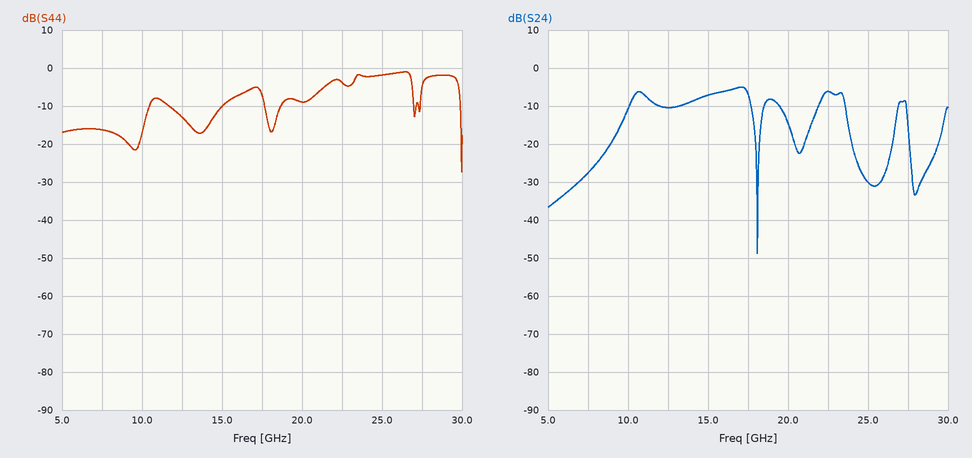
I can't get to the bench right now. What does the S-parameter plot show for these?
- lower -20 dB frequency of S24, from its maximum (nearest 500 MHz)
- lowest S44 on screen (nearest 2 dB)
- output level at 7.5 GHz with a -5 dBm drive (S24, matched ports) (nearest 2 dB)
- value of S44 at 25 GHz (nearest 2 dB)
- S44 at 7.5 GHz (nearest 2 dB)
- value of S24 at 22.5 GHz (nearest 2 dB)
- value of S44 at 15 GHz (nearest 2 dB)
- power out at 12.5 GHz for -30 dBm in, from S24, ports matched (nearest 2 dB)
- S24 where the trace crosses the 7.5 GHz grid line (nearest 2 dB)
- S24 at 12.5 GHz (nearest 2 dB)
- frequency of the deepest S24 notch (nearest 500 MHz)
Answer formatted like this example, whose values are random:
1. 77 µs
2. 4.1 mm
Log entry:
1. 8.0 GHz
2. -28 dB
3. -32 dBm
4. -2 dB
5. -16 dB
6. -6 dB
7. -10 dB
8. -40 dBm
9. -28 dB
10. -10 dB
11. 18.0 GHz
